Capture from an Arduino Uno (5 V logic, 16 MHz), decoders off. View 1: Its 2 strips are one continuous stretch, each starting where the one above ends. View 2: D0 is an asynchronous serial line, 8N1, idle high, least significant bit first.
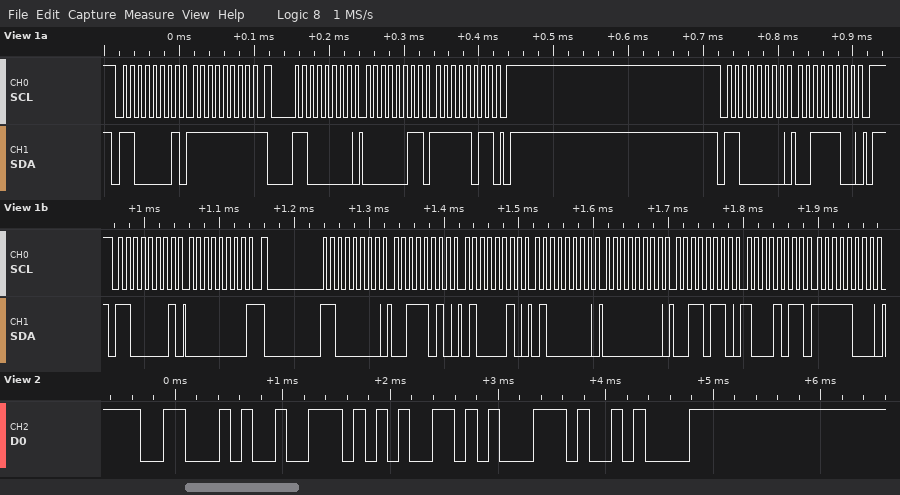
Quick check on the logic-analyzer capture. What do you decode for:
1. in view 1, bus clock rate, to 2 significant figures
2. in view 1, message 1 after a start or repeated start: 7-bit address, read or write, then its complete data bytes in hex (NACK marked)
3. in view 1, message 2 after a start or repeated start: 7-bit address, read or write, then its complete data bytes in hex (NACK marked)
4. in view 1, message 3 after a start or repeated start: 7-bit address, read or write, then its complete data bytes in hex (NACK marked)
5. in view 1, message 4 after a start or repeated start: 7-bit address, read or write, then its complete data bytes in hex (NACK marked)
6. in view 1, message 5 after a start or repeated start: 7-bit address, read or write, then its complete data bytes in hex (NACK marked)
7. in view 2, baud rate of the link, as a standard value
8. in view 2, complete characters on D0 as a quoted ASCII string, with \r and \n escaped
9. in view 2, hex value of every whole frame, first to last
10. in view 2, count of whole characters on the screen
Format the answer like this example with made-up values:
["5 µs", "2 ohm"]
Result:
["100 kHz", "0x60 read: FF NACK", "0x60 write: 03 FB", "0x60 write: 3C", "0x60 read: 00 NACK", "0x60 write: 3A 42 40 00 36 8B F8", "9600 baud", "\"Freq\\n\"", "0x46 0x72 0x65 0x71 0x0A", "5"]
